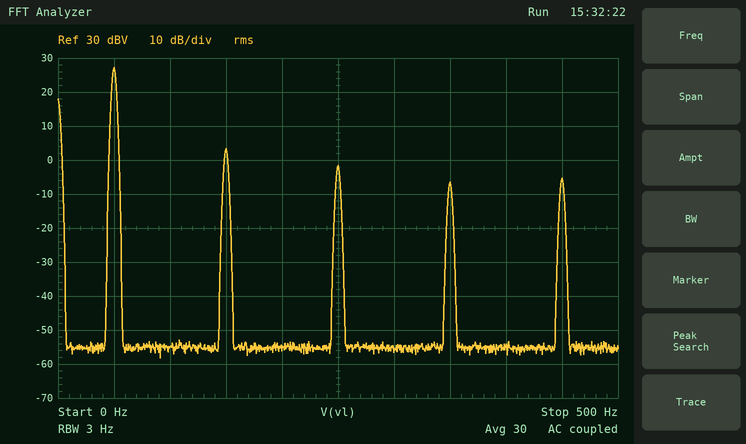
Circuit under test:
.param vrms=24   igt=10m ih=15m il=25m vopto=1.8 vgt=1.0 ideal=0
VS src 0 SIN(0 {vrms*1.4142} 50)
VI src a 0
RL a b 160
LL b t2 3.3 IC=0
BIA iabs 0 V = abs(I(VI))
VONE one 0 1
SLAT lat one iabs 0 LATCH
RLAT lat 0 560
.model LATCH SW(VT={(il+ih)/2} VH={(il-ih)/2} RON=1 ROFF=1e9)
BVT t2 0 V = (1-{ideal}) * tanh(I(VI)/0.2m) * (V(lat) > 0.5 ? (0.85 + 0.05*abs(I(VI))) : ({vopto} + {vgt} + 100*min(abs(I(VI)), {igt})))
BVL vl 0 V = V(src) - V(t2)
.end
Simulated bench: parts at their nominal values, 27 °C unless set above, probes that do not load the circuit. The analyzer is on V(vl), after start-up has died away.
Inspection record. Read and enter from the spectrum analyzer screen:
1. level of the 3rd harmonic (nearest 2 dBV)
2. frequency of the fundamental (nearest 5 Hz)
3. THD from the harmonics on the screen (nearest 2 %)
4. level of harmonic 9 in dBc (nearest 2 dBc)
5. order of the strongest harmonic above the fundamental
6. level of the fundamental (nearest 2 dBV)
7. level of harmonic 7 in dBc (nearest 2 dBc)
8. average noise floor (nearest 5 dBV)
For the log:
4 dBV
50 Hz
8 %
-32 dBc
3
28 dBV
-34 dBc
-55 dBV
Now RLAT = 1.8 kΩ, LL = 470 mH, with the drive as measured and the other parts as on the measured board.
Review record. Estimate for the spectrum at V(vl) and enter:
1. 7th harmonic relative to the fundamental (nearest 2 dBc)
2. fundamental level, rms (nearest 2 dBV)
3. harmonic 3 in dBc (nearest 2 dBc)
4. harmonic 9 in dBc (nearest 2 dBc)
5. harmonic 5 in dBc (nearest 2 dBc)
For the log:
-38 dBc
28 dBV
-36 dBc
-38 dBc
-38 dBc
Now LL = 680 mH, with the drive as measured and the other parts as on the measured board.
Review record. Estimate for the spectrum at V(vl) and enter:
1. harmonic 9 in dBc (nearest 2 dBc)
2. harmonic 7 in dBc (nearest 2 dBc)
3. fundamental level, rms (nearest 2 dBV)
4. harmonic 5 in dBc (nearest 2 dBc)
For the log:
-36 dBc
-36 dBc
28 dBV
-36 dBc
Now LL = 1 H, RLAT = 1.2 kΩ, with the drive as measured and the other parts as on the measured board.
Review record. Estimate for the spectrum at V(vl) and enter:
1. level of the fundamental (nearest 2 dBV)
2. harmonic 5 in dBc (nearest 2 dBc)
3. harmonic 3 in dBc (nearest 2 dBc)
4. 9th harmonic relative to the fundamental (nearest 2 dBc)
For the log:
28 dBV
-34 dBc
-34 dBc
-34 dBc
